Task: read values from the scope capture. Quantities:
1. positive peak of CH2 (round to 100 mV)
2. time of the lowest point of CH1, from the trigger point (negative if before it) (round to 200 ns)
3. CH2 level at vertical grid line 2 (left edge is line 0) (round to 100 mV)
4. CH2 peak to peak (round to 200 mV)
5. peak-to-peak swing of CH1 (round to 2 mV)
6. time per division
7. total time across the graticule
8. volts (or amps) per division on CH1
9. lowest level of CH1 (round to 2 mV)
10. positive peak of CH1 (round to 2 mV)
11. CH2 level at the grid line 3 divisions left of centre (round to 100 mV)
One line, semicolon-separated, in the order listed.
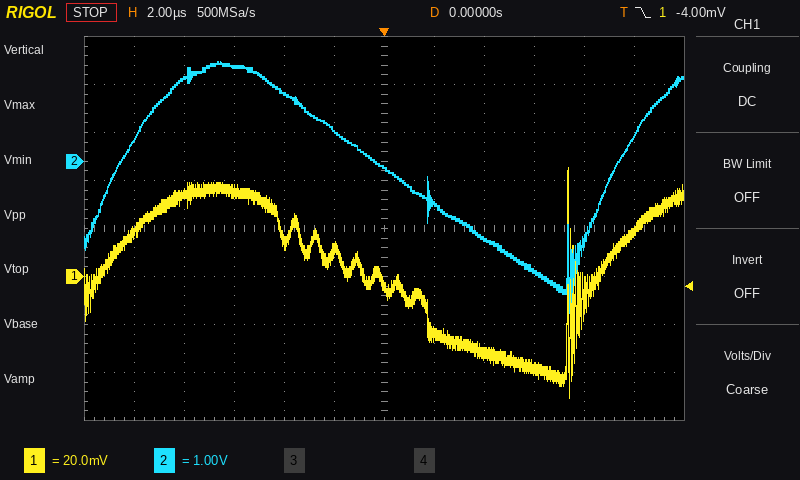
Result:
2.1 V; +7.4 µs; 1.7 V; 5.2 V; 96 mV; 2 µs; 24 µs; 20 mV; -50 mV; 46 mV; 2.0 V
